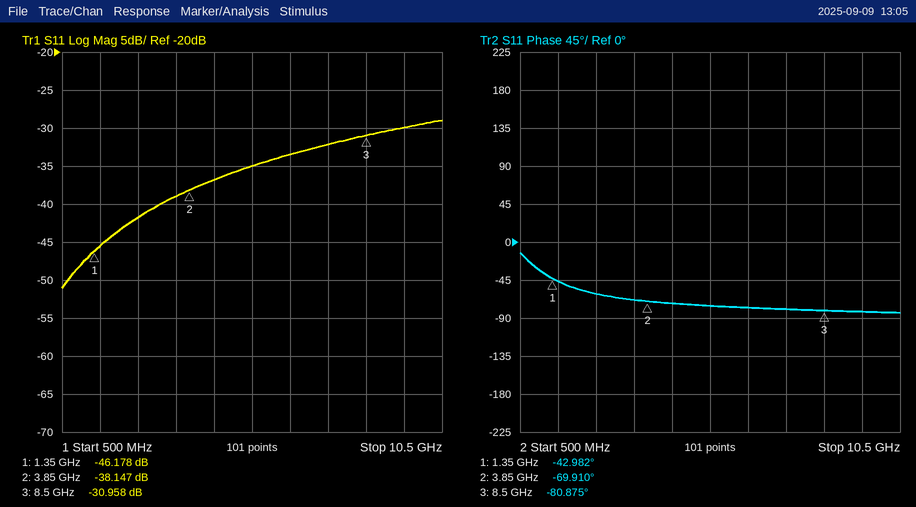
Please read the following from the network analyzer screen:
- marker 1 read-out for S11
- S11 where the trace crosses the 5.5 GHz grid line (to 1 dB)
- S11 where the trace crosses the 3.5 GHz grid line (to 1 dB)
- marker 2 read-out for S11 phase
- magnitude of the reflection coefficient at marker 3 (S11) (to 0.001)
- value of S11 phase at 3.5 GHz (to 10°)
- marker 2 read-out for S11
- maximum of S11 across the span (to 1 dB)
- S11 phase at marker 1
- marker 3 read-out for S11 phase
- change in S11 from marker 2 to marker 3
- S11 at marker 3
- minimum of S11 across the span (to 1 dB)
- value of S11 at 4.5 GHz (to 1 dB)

-46.178 dB
-35 dB
-39 dB
-69.910°
0.028
-70°
-38.147 dB
-29 dB
-42.982°
-80.875°
7.189 dB
-30.958 dB
-51 dB
-37 dB
